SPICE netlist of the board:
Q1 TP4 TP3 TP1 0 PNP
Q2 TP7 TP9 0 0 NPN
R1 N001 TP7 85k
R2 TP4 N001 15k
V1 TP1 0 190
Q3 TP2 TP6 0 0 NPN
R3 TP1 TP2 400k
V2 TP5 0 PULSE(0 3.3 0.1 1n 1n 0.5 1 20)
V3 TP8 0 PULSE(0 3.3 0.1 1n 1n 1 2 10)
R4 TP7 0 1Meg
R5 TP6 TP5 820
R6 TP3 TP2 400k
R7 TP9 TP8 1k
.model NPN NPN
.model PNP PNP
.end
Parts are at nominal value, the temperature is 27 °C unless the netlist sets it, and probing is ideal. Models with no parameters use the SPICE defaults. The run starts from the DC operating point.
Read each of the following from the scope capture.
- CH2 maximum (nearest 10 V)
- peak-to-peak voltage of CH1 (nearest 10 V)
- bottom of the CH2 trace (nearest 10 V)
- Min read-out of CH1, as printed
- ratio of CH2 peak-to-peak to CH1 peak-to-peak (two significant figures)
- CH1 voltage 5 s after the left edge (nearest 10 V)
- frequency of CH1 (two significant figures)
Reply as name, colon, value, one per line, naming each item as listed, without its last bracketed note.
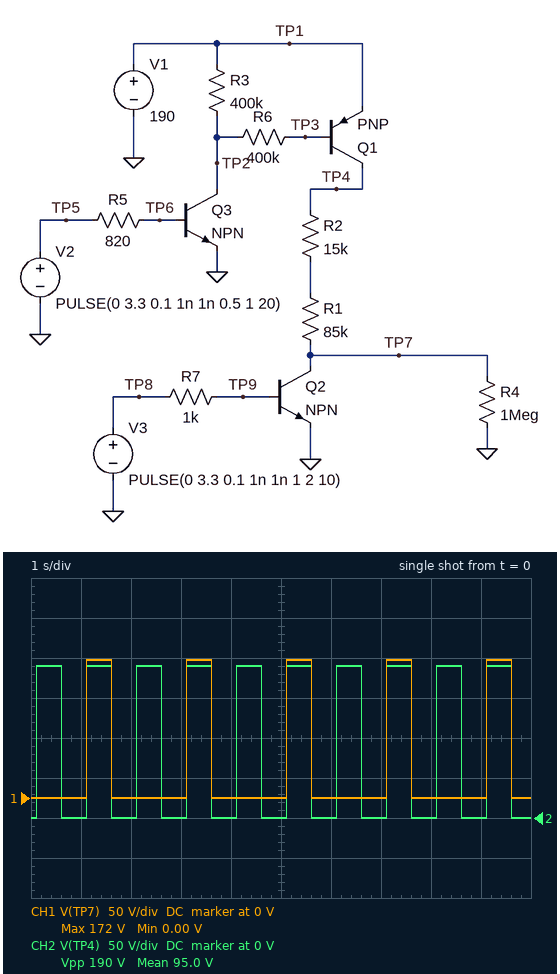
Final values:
CH2 maximum: 190 V
peak-to-peak voltage of CH1: 170 V
bottom of the CH2 trace: 0 V
Min read-out of CH1, as printed: 0.00 V
ratio of CH2 peak-to-peak to CH1 peak-to-peak: 1.1
CH1 voltage 5 s after the left edge: 0 V
frequency of CH1: 500 mHz
